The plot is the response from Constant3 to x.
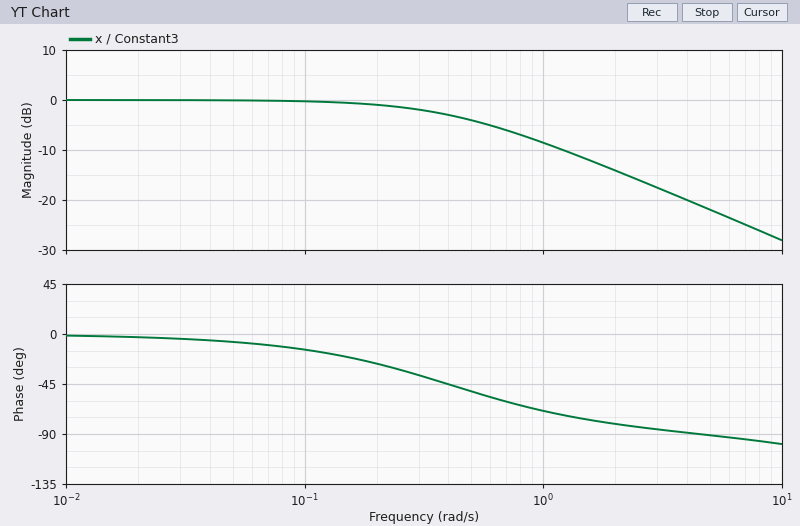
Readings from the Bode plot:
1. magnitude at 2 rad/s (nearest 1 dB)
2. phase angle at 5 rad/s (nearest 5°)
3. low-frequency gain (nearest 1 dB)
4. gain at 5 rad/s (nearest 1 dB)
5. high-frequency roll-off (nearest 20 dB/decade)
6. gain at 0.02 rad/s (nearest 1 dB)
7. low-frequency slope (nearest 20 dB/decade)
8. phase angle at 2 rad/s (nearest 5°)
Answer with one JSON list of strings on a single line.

["-14 dB", "-90°", "0 dB", "-22 dB", "-20 dB/decade", "0 dB", "0 dB/decade", "-80°"]
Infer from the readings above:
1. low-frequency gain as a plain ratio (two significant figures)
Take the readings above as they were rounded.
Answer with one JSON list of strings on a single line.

["1.0"]
